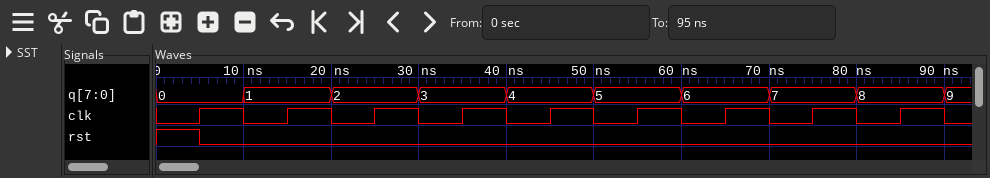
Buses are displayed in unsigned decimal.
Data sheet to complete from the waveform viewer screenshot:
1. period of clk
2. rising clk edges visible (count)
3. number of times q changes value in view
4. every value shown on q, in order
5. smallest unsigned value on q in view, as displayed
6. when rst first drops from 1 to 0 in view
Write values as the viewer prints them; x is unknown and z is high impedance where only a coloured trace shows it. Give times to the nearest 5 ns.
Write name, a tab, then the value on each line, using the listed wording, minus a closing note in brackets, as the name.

period of clk	10 ns
rising clk edges visible	9
number of times q changes value in view	9
every value shown on q, in order	0, 1, 2, 3, 4, 5, 6, 7, 8, 9
smallest unsigned value on q in view, as displayed	0
when rst first drops from 1 to 0 in view	5 ns
